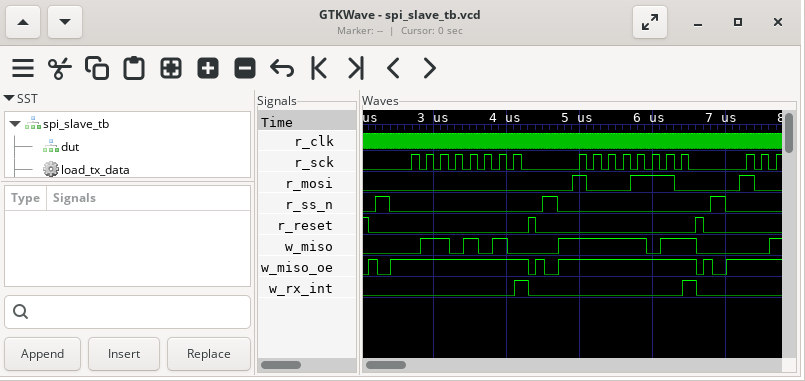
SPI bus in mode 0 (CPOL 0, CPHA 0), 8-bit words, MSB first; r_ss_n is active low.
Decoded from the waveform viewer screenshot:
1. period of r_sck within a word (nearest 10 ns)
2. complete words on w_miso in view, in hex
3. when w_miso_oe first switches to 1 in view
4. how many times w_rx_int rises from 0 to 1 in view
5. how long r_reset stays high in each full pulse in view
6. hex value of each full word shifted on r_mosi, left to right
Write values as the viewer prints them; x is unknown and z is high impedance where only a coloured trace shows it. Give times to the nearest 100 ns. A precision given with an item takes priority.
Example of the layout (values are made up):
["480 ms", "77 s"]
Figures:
["200 ns", "6A, FB", "2100 ns", "2", "100 ns, 100 ns", "00, 8E"]
